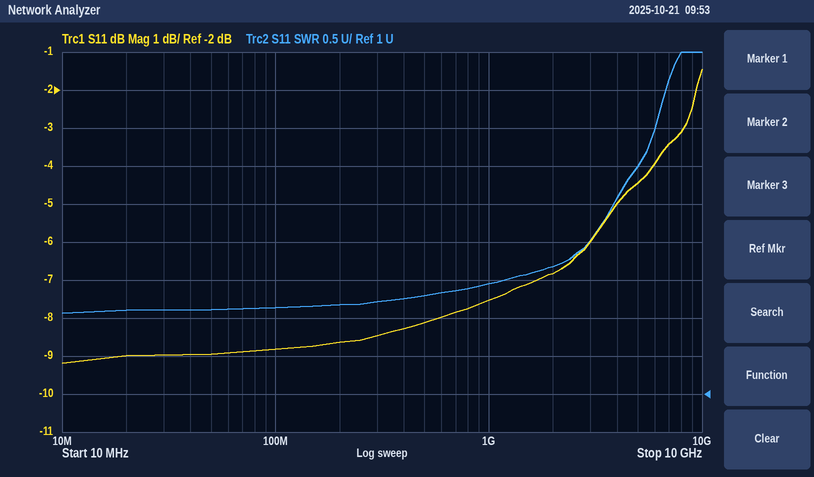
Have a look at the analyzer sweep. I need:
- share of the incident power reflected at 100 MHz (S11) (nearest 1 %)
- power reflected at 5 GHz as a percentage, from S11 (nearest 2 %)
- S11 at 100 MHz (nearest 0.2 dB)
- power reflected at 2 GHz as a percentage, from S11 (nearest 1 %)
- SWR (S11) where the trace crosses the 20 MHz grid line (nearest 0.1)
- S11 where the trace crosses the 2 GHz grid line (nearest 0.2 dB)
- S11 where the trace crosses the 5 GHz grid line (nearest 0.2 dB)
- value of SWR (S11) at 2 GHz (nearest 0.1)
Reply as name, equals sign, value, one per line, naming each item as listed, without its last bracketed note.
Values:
share of the incident power reflected at 100 MHz (S11) = 13 %
power reflected at 5 GHz as a percentage, from S11 = 36 %
S11 at 100 MHz = -8.8 dB
power reflected at 2 GHz as a percentage, from S11 = 21 %
SWR (S11) where the trace crosses the 20 MHz grid line = 2.1
S11 where the trace crosses the 2 GHz grid line = -6.8 dB
S11 where the trace crosses the 5 GHz grid line = -4.4 dB
value of SWR (S11) at 2 GHz = 2.7
